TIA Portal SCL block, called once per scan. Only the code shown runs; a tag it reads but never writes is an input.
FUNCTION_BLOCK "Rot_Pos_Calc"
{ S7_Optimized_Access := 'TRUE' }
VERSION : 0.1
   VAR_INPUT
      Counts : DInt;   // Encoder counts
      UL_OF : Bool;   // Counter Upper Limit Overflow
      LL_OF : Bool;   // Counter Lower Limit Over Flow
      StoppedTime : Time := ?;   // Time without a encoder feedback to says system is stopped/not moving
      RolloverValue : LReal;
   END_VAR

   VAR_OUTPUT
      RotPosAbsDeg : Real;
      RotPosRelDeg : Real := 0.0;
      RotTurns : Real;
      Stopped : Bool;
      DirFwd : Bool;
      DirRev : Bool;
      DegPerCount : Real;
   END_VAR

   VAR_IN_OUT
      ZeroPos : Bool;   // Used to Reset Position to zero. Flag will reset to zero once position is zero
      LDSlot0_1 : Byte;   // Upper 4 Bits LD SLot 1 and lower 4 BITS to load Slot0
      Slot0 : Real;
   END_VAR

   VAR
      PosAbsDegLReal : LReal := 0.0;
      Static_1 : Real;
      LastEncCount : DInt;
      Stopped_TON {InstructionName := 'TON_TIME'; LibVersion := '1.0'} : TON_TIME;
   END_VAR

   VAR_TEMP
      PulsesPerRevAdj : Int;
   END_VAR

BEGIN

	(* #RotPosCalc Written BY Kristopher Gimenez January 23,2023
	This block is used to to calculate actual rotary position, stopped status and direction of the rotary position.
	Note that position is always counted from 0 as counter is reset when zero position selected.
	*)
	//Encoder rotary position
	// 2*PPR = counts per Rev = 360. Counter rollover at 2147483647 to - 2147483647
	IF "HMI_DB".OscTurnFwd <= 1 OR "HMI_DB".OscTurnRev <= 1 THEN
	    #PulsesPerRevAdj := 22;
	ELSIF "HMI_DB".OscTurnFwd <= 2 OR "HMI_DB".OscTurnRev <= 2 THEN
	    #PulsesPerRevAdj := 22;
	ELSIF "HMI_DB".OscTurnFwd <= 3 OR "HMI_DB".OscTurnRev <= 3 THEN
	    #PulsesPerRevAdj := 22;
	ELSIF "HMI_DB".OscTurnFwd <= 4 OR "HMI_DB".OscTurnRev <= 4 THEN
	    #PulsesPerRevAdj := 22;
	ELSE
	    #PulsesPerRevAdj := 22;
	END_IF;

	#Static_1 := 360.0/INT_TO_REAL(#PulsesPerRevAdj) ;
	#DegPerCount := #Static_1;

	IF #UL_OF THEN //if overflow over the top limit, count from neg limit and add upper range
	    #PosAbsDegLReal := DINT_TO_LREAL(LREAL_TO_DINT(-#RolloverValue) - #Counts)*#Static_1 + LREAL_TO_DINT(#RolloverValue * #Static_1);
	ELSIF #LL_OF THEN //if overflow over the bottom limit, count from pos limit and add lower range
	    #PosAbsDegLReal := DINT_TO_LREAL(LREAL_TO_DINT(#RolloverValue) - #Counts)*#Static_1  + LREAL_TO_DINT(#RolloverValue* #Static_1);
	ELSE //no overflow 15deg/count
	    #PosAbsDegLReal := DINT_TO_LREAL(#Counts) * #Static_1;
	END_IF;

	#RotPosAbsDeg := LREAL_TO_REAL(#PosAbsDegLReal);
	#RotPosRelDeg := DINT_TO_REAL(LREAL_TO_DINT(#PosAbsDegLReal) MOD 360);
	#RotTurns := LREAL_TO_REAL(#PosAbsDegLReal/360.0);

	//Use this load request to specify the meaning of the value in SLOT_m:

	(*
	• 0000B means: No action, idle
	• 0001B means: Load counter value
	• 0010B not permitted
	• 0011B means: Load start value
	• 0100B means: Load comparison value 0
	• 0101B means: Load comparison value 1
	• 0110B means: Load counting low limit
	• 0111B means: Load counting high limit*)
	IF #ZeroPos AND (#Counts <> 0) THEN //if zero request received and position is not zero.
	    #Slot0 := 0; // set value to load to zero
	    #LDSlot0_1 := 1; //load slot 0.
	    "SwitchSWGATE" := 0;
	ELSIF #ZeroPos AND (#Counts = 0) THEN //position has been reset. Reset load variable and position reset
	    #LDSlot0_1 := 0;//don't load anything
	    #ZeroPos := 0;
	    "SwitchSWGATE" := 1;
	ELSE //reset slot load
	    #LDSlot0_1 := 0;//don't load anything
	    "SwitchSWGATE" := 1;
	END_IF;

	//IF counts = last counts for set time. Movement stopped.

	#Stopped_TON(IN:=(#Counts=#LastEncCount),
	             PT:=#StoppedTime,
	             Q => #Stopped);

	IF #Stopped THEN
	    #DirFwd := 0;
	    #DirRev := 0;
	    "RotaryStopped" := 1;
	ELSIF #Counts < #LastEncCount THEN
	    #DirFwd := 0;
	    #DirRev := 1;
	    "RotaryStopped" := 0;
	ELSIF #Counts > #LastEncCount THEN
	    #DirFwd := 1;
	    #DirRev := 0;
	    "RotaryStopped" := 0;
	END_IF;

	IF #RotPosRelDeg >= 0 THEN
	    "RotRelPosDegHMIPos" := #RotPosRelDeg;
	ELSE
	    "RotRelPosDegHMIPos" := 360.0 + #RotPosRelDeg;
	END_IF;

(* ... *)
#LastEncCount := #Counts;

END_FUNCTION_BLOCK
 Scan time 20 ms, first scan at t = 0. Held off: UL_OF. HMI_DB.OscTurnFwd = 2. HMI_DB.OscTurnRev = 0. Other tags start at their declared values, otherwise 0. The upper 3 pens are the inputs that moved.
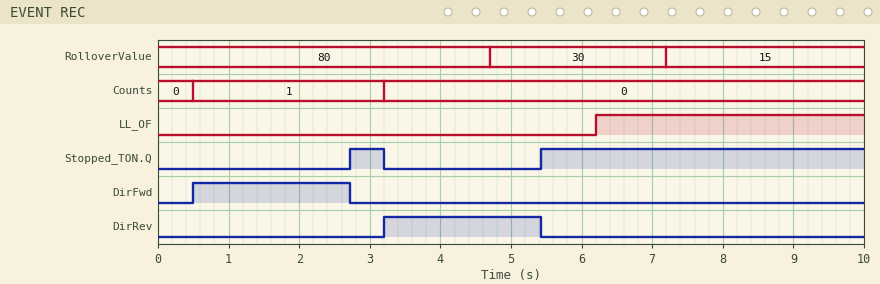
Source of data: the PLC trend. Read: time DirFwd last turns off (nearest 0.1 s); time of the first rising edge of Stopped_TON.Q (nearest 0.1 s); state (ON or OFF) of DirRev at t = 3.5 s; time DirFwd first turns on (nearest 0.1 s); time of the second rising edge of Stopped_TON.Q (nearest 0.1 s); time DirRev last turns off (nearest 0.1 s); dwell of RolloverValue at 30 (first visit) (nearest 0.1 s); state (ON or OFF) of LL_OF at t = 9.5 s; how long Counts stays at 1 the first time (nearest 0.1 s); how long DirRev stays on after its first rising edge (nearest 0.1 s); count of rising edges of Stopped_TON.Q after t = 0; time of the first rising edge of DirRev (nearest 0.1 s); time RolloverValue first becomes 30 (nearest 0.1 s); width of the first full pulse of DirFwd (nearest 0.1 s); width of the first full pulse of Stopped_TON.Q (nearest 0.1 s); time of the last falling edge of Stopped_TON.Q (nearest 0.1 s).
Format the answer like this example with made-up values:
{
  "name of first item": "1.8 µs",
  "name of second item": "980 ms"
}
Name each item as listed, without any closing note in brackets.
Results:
{
  "time DirFwd last turns off": "2.7 s",
  "time of the first rising edge of Stopped_TON.Q": "2.7 s",
  "state (ON or OFF) of DirRev at t = 3.5 s": "ON",
  "time DirFwd first turns on": "0.5 s",
  "time of the second rising edge of Stopped_TON.Q": "5.4 s",
  "time DirRev last turns off": "5.4 s",
  "dwell of RolloverValue at 30 (first visit)": "2.5 s",
  "state (ON or OFF) of LL_OF at t = 9.5 s": "ON",
  "how long Counts stays at 1 the first time": "2.7 s",
  "how long DirRev stays on after its first rising edge": "2.2 s",
  "count of rising edges of Stopped_TON.Q after t = 0": "2",
  "time of the first rising edge of DirRev": "3.2 s",
  "time RolloverValue first becomes 30": "4.7 s",
  "width of the first full pulse of DirFwd": "2.2 s",
  "width of the first full pulse of Stopped_TON.Q": "0.5 s",
  "time of the last falling edge of Stopped_TON.Q": "3.2 s"
}
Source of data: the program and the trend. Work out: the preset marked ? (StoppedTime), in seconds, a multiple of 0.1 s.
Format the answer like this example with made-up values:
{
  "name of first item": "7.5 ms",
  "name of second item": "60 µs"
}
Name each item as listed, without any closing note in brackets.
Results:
{
  "the preset marked ? (StoppedTime), in seconds, a multiple of 0.1 s": "2.2 s"
}
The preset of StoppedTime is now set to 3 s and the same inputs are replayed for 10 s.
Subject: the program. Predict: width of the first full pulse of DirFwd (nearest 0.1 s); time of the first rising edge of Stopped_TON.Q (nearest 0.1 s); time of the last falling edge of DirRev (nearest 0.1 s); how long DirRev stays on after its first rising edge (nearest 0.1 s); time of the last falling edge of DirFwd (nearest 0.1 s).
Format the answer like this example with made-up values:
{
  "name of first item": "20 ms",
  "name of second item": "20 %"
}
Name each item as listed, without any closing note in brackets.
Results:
{
  "width of the first full pulse of DirFwd": "2.7 s",
  "time of the first rising edge of Stopped_TON.Q": "6.2 s",
  "time of the last falling edge of DirRev": "6.2 s",
  "how long DirRev stays on after its first rising edge": "3.0 s",
  "time of the last falling edge of DirFwd": "3.2 s"
}
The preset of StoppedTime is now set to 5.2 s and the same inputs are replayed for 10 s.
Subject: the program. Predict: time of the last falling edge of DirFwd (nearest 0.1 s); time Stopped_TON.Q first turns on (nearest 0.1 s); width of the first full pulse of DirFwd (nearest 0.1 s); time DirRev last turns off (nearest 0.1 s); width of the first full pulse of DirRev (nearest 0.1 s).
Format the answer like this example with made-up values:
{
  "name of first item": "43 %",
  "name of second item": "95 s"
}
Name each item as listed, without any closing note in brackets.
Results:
{
  "time of the last falling edge of DirFwd": "3.2 s",
  "time Stopped_TON.Q first turns on": "8.4 s",
  "width of the first full pulse of DirFwd": "2.7 s",
  "time DirRev last turns off": "8.4 s",
  "width of the first full pulse of DirRev": "5.2 s"
}
